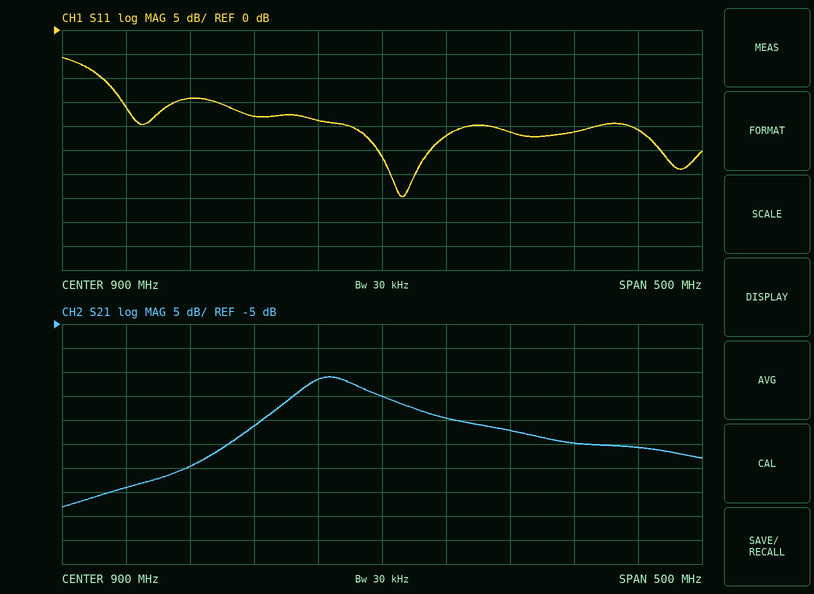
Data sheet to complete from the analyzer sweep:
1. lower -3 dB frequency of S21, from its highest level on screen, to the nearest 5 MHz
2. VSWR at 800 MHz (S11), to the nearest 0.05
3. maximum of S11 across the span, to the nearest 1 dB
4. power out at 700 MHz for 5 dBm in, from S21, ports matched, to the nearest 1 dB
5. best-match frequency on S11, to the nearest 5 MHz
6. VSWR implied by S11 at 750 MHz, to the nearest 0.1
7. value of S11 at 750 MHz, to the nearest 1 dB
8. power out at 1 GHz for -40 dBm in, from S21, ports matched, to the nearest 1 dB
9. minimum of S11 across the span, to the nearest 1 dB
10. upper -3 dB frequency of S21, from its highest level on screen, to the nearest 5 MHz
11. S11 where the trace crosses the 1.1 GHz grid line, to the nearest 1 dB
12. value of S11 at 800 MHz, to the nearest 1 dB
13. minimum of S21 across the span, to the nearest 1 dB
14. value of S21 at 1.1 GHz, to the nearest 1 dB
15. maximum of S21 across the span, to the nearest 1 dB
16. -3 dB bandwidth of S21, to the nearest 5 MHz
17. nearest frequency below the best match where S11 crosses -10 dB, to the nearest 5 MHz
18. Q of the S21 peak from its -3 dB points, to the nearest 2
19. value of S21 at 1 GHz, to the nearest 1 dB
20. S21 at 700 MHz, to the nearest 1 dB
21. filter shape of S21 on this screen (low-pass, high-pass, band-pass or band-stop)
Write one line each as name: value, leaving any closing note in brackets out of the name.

lower -3 dB frequency of S21, from its highest level on screen, to the nearest 5 MHz: 835 MHz
VSWR at 800 MHz (S11), to the nearest 0.05: 1.30
maximum of S11 across the span, to the nearest 1 dB: -6 dB
power out at 700 MHz for 5 dBm in, from S21, ports matched, to the nearest 1 dB: -34 dBm
best-match frequency on S11, to the nearest 5 MHz: 915 MHz
VSWR implied by S11 at 750 MHz, to the nearest 0.1: 1.5
value of S11 at 750 MHz, to the nearest 1 dB: -14 dB
power out at 1 GHz for -40 dBm in, from S21, ports matched, to the nearest 1 dB: -67 dBm
minimum of S11 across the span, to the nearest 1 dB: -35 dB
upper -3 dB frequency of S21, from its highest level on screen, to the nearest 5 MHz: 890 MHz
S11 where the trace crosses the 1.1 GHz grid line, to the nearest 1 dB: -21 dB
value of S11 at 800 MHz, to the nearest 1 dB: -18 dB
minimum of S21 across the span, to the nearest 1 dB: -43 dB
value of S21 at 1.1 GHz, to the nearest 1 dB: -31 dB
maximum of S21 across the span, to the nearest 1 dB: -16 dB
-3 dB bandwidth of S21, to the nearest 5 MHz: 55 MHz
nearest frequency below the best match where S11 crosses -10 dB, to the nearest 5 MHz: 680 MHz
Q of the S21 peak from its -3 dB points, to the nearest 2: 16
value of S21 at 1 GHz, to the nearest 1 dB: -27 dB
S21 at 700 MHz, to the nearest 1 dB: -39 dB
filter shape of S21 on this screen: band-pass
